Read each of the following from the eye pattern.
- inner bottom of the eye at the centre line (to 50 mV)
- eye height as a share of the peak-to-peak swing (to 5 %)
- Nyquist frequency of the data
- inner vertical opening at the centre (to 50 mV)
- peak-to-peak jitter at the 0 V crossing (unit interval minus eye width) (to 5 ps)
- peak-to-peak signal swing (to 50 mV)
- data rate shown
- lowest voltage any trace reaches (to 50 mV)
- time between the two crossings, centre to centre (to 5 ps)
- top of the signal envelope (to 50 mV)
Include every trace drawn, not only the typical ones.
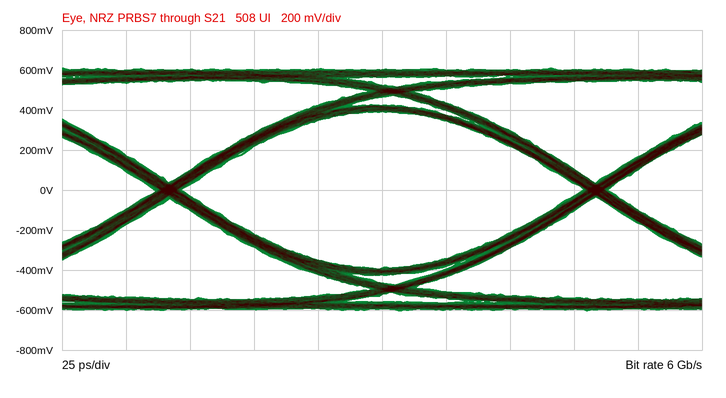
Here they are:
-400 mV
65 %
3 GHz
800 mV
10 ps
1.20 V
6 Gb/s
-600 mV
165 ps
600 mV
